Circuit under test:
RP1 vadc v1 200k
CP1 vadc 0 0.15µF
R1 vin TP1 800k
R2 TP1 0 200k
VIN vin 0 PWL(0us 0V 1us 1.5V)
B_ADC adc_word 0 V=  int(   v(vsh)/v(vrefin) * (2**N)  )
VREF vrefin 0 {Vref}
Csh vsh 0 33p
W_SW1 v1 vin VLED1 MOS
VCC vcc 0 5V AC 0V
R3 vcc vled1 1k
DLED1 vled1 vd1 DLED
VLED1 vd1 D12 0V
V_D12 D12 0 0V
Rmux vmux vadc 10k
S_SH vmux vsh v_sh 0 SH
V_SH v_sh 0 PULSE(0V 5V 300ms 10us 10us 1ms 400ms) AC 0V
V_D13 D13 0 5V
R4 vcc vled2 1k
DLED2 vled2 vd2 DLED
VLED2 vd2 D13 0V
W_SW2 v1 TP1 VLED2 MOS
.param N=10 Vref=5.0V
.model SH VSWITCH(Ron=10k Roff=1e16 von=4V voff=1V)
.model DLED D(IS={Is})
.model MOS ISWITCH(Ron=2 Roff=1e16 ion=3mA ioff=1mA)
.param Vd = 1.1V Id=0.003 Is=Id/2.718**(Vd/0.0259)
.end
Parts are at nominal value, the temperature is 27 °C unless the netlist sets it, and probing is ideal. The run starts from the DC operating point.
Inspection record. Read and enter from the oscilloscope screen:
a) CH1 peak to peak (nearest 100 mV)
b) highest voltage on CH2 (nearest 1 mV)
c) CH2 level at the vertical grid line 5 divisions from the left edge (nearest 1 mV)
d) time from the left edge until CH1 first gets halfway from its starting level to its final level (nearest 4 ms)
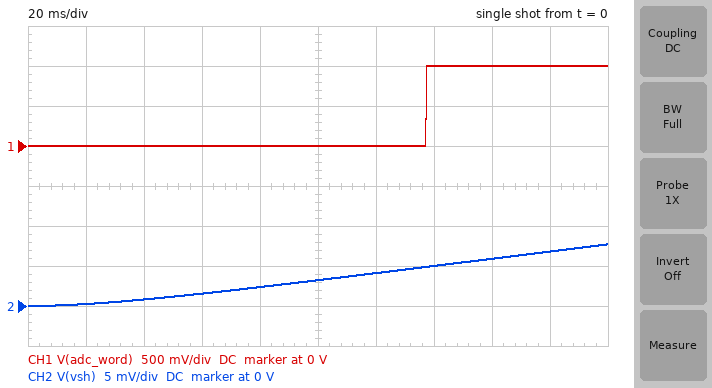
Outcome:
1.0 V
8 mV
3 mV
136 ms
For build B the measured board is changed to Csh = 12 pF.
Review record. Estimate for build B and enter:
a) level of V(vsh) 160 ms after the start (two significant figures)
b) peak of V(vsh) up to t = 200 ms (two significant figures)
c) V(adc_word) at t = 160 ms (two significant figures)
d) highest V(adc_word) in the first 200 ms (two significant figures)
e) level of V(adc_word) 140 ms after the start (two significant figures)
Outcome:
16 mV
21 mV
3.0 V
4.0 V
2.0 V
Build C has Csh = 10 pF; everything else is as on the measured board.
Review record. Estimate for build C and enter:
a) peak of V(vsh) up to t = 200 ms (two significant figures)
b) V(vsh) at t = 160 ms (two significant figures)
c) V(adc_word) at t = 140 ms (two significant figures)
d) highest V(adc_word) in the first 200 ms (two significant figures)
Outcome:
25 mV
19 mV
3.0 V
5.0 V
